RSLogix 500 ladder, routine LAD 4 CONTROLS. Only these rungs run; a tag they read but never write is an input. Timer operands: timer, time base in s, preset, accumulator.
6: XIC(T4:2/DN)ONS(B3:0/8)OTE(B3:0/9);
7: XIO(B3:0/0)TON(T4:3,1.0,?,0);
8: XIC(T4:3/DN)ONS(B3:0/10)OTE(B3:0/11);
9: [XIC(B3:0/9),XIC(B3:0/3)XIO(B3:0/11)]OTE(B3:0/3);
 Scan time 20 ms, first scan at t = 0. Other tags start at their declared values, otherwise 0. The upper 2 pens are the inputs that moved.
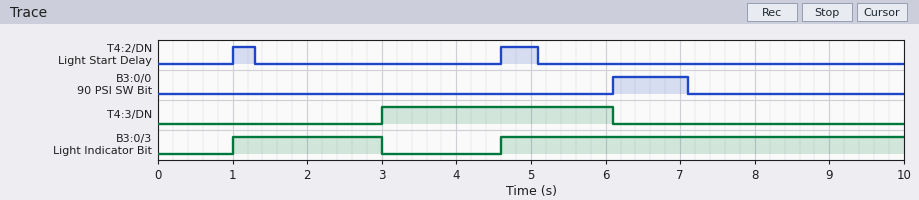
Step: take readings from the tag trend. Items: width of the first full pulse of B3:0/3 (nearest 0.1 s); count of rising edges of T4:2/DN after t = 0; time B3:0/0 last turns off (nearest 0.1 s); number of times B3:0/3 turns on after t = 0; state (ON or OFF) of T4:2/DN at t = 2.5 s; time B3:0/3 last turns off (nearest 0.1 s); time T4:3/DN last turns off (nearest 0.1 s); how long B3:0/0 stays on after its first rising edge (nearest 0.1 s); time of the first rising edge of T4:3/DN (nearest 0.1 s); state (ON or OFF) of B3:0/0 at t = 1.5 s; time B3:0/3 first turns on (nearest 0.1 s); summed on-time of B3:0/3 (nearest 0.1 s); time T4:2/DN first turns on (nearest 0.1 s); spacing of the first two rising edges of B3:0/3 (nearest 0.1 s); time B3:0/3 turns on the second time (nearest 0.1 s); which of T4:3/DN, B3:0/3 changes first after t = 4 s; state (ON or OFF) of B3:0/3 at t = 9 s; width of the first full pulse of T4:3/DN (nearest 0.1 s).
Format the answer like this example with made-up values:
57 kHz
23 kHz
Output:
2.0 s
2
7.1 s
2
OFF
3.0 s
6.1 s
1.0 s
3.0 s
OFF
1.0 s
7.4 s
1.0 s
3.6 s
4.6 s
B3:0/3
ON
3.1 s
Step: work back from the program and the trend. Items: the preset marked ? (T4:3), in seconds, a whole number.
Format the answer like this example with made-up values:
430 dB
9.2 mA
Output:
3 s
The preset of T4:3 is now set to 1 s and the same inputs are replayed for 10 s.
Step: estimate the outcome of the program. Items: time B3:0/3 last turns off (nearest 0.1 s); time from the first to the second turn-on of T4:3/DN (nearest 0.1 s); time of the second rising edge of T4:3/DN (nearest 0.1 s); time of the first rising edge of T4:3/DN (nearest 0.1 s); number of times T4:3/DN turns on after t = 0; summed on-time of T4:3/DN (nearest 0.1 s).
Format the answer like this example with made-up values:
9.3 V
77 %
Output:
8.1 s
7.1 s
8.1 s
1.0 s
2
7.0 s
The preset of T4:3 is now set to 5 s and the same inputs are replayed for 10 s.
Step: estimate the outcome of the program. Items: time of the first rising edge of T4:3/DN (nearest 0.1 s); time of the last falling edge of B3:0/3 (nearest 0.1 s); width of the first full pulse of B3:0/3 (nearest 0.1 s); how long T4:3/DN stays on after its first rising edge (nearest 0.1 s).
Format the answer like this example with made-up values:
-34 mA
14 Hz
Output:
5.0 s
5.0 s
4.0 s
1.1 s
